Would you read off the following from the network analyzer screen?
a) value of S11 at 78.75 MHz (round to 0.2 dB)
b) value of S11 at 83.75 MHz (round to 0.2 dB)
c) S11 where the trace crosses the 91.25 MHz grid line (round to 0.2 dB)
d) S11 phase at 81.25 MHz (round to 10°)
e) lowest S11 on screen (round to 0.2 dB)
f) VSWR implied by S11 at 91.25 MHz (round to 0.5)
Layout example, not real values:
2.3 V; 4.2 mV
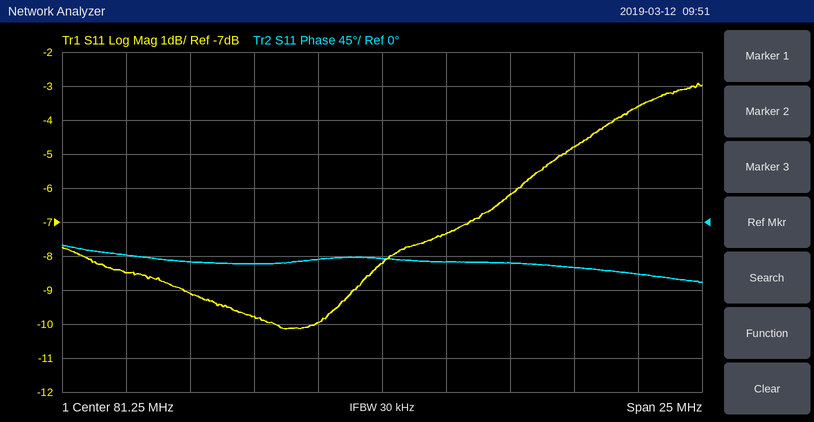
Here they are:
-10.0 dB; -7.4 dB; -3.6 dB; -50°; -10.2 dB; 5.0
